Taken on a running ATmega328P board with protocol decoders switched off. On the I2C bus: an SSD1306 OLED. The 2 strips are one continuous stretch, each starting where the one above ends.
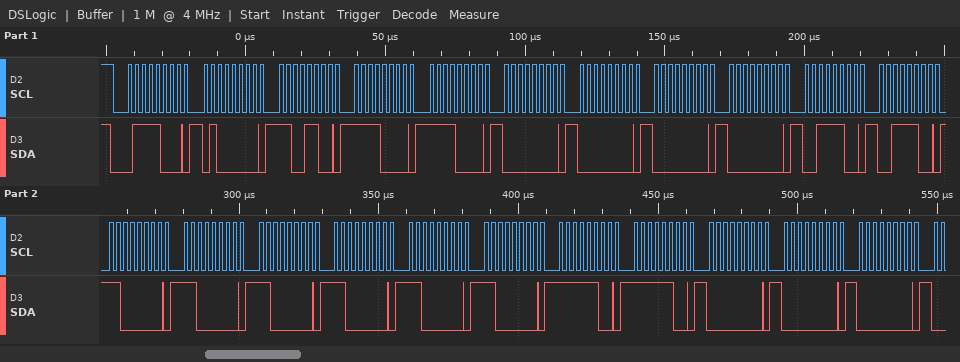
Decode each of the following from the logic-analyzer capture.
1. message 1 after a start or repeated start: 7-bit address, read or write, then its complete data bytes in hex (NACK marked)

0x3C write: 40 CC F0 F0 00 00 00 00 3C 3C C0 C0 C0 C0 C0 C0 FC FC 00 00 00
